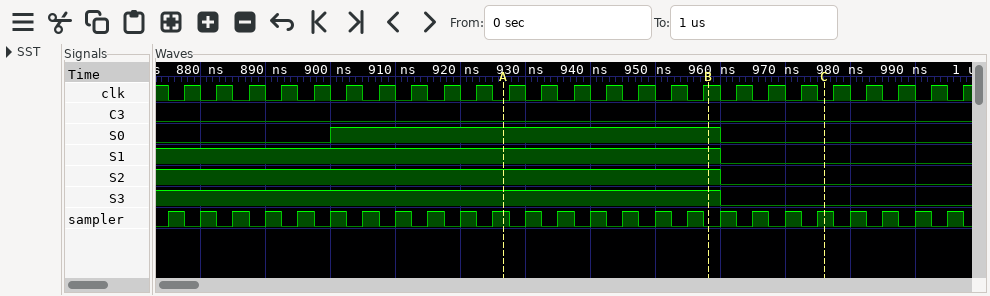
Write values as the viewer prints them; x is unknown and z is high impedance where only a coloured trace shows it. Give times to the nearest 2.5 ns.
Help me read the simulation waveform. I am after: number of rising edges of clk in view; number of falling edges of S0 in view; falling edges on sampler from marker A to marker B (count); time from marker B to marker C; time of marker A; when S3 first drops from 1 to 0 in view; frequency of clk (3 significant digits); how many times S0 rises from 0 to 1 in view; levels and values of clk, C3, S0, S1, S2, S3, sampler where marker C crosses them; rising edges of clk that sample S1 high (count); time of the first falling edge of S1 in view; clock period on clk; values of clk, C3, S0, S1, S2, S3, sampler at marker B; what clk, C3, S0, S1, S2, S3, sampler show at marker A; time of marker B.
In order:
25
1
7
17.5 ns
927.5 ns
960 ns
200 MHz
1
clk=0, C3=0, S0=0, S1=0, S2=0, S3=0, sampler=1
17
960 ns
5 ns
clk=1, C3=0, S0=1, S1=1, S2=1, S3=1, sampler=0
clk=0, C3=0, S0=1, S1=1, S2=1, S3=1, sampler=1
957.5 ns
